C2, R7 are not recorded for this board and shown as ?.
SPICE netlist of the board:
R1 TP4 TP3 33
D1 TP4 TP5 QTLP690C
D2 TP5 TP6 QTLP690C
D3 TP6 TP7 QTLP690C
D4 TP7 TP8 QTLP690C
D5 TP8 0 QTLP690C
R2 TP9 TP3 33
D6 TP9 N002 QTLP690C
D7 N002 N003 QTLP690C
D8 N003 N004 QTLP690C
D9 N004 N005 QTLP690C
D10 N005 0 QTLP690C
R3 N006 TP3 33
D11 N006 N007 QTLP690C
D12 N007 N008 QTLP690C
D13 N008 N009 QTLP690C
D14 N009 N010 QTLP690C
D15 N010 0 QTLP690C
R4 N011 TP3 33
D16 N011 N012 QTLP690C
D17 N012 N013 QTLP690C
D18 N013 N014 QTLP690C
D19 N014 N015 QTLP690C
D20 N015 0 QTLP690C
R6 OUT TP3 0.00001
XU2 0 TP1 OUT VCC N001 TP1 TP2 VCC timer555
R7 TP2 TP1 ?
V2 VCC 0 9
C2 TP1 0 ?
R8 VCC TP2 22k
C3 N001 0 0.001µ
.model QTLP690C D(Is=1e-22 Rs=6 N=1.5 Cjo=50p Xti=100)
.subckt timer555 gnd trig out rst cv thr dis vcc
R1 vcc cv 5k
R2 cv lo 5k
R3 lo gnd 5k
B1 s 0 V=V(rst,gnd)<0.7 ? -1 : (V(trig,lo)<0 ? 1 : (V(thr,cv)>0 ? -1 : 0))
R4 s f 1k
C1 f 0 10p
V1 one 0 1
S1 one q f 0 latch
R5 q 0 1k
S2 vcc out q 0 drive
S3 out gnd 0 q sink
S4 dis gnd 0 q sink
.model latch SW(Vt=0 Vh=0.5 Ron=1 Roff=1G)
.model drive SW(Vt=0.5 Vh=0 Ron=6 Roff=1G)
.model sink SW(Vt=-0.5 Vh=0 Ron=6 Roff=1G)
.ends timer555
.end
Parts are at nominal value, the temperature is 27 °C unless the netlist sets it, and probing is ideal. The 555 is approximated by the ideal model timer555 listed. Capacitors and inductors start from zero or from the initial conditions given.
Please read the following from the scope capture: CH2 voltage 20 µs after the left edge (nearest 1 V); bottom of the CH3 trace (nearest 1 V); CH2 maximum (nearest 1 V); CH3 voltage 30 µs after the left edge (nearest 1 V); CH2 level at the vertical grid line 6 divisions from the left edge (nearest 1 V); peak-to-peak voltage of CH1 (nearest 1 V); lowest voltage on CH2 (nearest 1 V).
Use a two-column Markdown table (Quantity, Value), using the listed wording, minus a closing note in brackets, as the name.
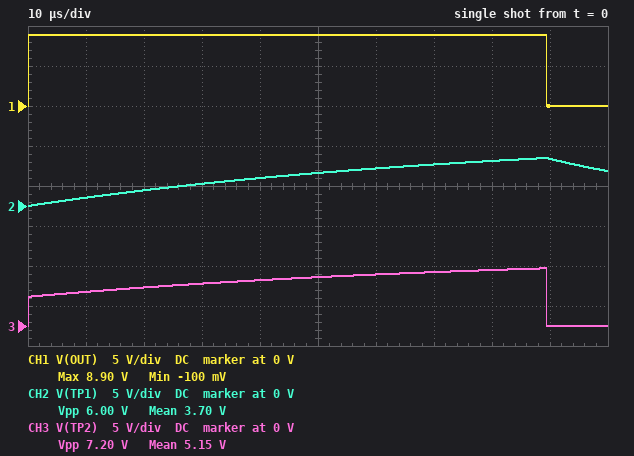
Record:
| Quantity | Value |
|---|---|
| CH2 voltage 20 µs after the left edge | 2 V |
| bottom of the CH3 trace | 0 V |
| CH2 maximum | 6 V |
| CH3 voltage 30 µs after the left edge | 5 V |
| CH2 level at the vertical grid line 6 divisions from the left edge | 5 V |
| peak-to-peak voltage of CH1 | 9 V |
| lowest voltage on CH2 | 0 V |
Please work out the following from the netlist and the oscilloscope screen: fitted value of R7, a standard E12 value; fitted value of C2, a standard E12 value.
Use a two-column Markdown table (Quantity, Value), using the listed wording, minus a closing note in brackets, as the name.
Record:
| Quantity | Value |
|---|---|
| fitted value of R7, a standard E12 value | 15 kΩ |
| fitted value of C2, a standard E12 value | 2.2 nF |
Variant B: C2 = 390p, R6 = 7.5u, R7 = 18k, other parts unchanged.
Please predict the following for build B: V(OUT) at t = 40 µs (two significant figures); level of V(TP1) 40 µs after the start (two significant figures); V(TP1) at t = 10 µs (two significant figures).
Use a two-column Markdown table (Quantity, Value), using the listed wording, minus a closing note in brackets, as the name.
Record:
| Quantity | Value |
|---|---|
| V(OUT) at t = 40 µs | 8.9 V |
| level of V(TP1) 40 µs after the start | 3.9 V |
| V(TP1) at t = 10 µs | 4.3 V |
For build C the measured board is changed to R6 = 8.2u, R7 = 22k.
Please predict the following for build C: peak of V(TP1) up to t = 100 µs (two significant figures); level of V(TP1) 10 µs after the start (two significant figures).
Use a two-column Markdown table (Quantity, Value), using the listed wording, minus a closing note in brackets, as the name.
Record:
| Quantity | Value |
|---|---|
| peak of V(TP1) up to t = 100 µs | 5.8 V |
| level of V(TP1) 10 µs after the start | 880 mV |
